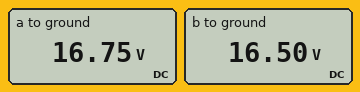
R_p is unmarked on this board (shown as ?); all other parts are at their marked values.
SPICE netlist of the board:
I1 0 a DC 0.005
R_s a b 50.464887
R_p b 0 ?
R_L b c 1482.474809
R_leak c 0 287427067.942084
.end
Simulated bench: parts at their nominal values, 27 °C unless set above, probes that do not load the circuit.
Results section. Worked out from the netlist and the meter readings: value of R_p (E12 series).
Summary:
3.3 kΩ
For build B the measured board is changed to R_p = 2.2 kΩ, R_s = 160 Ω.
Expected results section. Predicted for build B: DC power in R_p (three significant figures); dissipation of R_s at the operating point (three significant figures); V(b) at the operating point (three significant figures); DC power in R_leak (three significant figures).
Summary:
55.0 mW
4.00 mW
11.0 V
421 nW
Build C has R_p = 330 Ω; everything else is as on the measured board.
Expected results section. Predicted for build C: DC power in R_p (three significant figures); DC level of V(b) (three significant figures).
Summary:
8.25 mW
1.65 V
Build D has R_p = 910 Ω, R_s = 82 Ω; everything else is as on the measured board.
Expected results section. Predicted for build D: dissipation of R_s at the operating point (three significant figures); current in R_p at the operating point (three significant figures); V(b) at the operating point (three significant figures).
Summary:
2.05 mW
5.00 mA
4.55 V
